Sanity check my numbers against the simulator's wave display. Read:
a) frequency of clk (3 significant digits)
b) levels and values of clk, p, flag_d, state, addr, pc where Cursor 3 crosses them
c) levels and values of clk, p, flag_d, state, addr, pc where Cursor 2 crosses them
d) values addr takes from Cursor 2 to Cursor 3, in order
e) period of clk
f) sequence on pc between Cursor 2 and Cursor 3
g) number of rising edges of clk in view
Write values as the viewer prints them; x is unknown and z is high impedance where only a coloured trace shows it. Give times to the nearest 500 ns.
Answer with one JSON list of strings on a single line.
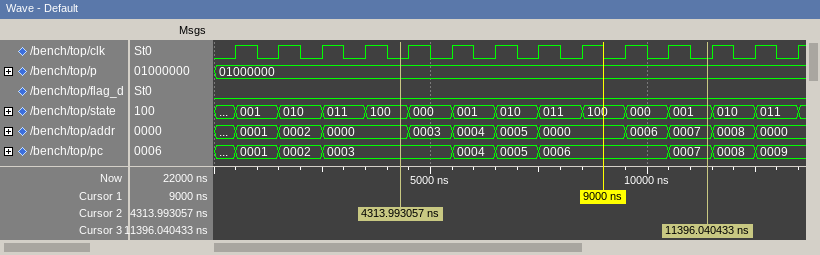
["1.00 MHz", "clk=0, p=01000000, flag_d=0, state=001, addr=0007, pc=0007", "clk=0, p=01000000, flag_d=0, state=100, addr=0000, pc=0003", "0000, 0003, 0004, 0005, 0000, 0006, 0007", "1000 ns", "0003, 0004, 0005, 0006, 0007", "14"]
